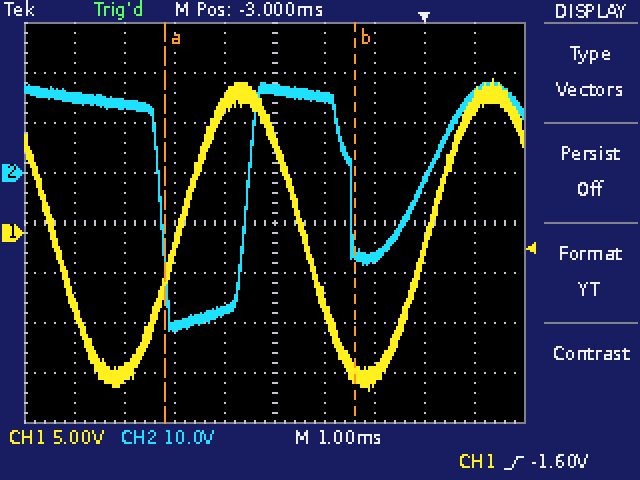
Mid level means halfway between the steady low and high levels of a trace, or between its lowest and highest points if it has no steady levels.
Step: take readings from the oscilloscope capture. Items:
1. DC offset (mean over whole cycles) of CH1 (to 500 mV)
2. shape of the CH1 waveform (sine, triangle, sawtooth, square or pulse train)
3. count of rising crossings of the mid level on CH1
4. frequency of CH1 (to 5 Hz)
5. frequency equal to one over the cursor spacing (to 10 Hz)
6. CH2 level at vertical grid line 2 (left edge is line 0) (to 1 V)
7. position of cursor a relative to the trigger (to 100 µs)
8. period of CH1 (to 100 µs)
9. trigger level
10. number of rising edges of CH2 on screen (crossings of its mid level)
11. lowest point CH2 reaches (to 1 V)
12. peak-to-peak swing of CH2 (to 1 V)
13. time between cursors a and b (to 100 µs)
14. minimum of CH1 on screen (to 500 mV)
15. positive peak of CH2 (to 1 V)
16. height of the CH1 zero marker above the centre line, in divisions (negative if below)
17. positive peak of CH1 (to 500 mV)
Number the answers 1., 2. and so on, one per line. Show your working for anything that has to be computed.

1. (15.5 V + (-16.0 V)) / 2 ≈ 0.0 V
2. sine
3. 2
4. 1 / 5.0 ms ≈ 200 Hz
5. 1 / 3.8 ms ≈ 260 Hz
6. 14 V
7. -5.2 ms
8. 5.0 ms
9. -1.60 V
10. 2
11. -32 V
12. 18 V − (-32 V) = 50 V
13. 3.8 ms
14. -16.0 V
15. 18 V
16. -0.2 div
17. 15.5 V
